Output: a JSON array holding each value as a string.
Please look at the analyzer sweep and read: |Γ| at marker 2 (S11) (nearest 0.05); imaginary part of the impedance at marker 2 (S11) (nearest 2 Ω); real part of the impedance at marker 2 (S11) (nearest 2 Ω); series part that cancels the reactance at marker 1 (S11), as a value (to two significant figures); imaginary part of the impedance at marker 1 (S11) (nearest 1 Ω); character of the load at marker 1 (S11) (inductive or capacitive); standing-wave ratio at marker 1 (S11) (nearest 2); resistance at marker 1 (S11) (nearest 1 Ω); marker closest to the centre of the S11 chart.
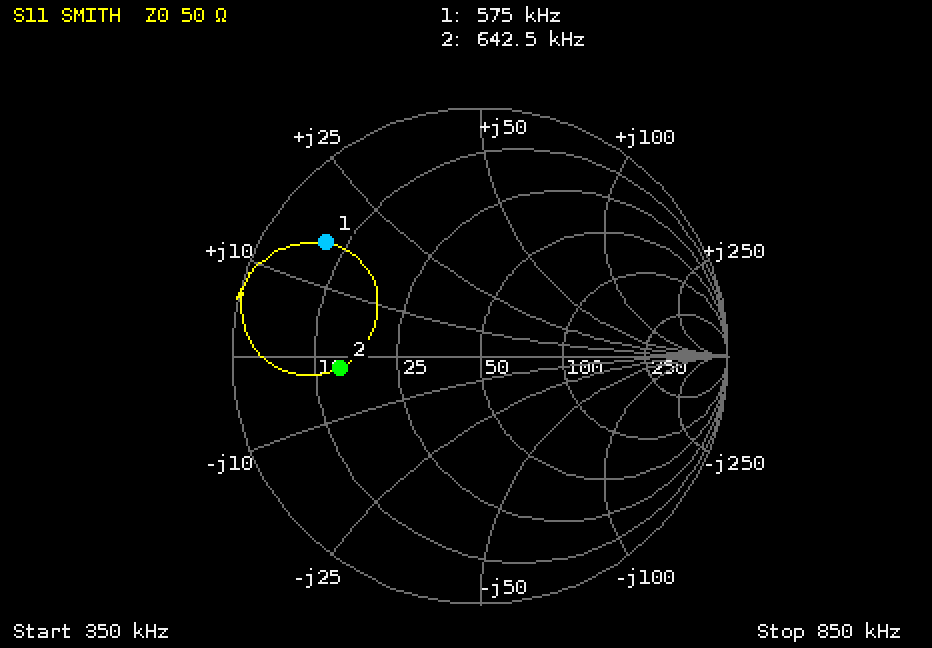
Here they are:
["0.55", "-2 Ω", "14 Ω", "17 nF", "+16 Ω", "inductive", "8", "7 Ω", "marker 2"]
